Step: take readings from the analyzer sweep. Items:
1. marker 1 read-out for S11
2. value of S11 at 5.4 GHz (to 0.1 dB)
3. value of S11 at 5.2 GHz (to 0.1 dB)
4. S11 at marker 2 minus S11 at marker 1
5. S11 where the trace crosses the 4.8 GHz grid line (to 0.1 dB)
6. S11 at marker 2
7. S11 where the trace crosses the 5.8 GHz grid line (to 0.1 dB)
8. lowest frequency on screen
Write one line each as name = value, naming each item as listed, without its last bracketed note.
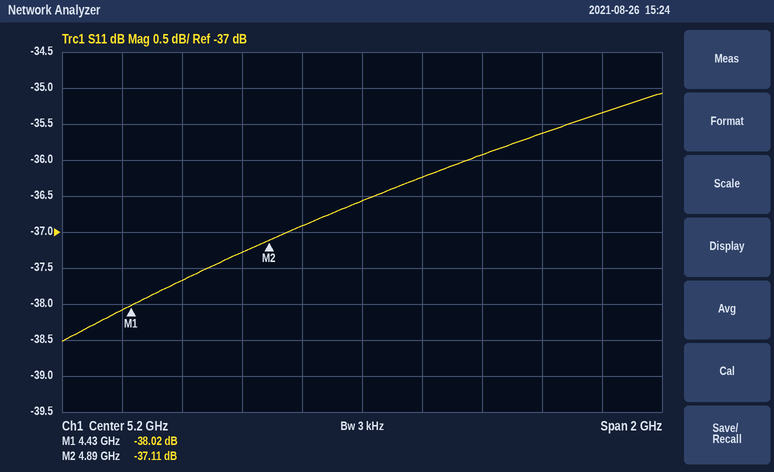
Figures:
marker 1 read-out for S11 = -38.02 dB
value of S11 at 5.4 GHz = -36.2 dB
value of S11 at 5.2 GHz = -36.6 dB
S11 at marker 2 minus S11 at marker 1 = 0.91 dB
S11 where the trace crosses the 4.8 GHz grid line = -37.3 dB
S11 at marker 2 = -37.11 dB
S11 where the trace crosses the 5.8 GHz grid line = -35.6 dB
lowest frequency on screen = 4.2 GHz
